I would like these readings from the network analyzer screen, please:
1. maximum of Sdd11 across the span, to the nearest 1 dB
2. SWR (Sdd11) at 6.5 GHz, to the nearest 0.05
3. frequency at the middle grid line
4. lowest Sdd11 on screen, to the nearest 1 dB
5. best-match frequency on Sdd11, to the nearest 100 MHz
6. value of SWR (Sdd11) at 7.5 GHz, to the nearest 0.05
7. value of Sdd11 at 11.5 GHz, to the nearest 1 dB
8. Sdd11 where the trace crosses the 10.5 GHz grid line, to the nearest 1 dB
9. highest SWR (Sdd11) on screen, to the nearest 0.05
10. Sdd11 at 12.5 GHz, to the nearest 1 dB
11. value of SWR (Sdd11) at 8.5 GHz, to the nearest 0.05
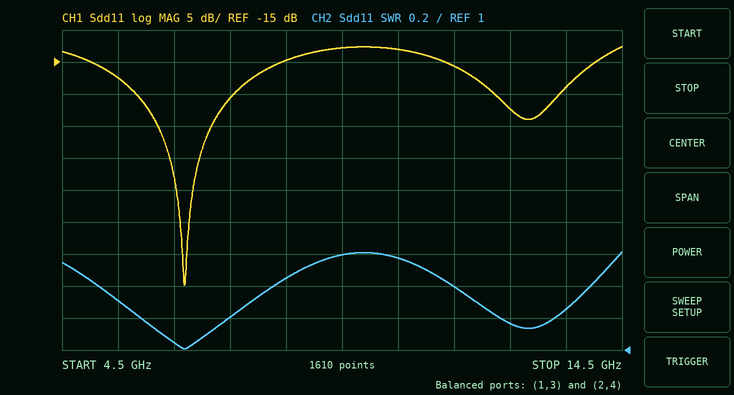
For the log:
-13 dB
1.05
9.5 GHz
-50 dB
6.7 GHz
1.20
-16 dB
-13 dB
1.60
-22 dB
1.45
